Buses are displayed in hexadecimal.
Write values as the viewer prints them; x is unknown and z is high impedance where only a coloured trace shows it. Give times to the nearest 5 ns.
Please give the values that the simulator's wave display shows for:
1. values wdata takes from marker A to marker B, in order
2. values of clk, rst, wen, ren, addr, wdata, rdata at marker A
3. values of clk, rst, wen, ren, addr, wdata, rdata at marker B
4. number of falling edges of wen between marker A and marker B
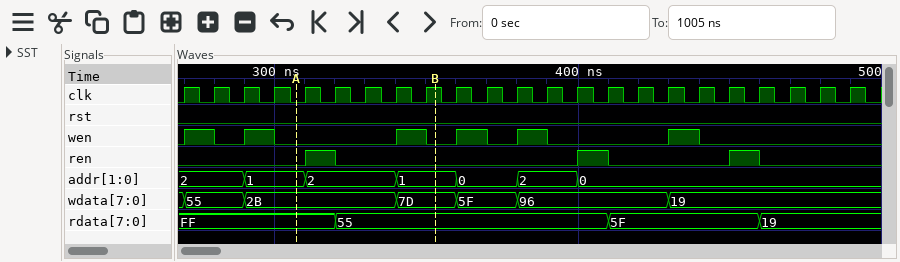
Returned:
2B, 7D
clk=0, rst=0, wen=0, ren=0, addr=1, wdata=2B, rdata=FF
clk=1, rst=0, wen=0, ren=0, addr=1, wdata=7D, rdata=55
1
